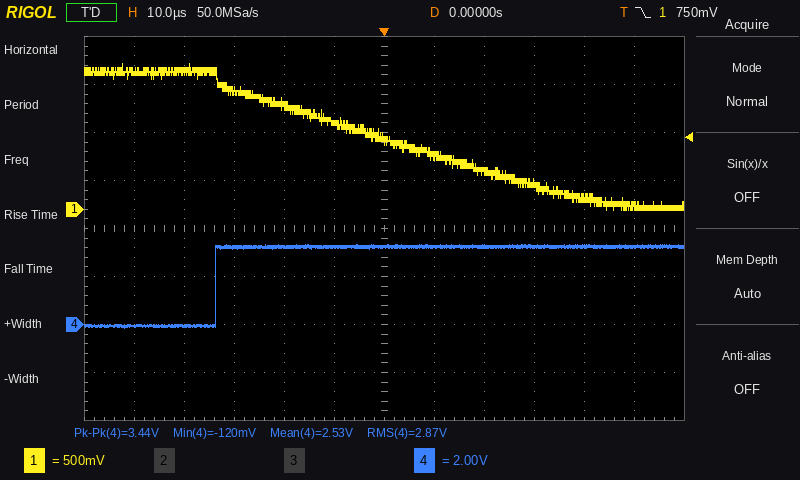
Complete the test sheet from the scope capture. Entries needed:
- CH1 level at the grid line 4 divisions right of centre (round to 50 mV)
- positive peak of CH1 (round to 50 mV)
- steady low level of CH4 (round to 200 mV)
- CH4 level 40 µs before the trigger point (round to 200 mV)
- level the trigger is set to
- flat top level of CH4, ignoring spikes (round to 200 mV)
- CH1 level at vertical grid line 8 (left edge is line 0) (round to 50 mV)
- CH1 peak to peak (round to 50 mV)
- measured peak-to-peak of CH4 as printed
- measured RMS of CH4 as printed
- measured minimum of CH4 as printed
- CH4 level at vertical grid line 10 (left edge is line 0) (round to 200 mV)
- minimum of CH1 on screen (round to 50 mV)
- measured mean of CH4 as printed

100 mV
1.50 V
0.0 V
0.0 V
750 mV
3.2 V
400 mV
1.50 V
3.44 V
2.87 V
-120 mV
3.2 V
0 mV
2.53 V
